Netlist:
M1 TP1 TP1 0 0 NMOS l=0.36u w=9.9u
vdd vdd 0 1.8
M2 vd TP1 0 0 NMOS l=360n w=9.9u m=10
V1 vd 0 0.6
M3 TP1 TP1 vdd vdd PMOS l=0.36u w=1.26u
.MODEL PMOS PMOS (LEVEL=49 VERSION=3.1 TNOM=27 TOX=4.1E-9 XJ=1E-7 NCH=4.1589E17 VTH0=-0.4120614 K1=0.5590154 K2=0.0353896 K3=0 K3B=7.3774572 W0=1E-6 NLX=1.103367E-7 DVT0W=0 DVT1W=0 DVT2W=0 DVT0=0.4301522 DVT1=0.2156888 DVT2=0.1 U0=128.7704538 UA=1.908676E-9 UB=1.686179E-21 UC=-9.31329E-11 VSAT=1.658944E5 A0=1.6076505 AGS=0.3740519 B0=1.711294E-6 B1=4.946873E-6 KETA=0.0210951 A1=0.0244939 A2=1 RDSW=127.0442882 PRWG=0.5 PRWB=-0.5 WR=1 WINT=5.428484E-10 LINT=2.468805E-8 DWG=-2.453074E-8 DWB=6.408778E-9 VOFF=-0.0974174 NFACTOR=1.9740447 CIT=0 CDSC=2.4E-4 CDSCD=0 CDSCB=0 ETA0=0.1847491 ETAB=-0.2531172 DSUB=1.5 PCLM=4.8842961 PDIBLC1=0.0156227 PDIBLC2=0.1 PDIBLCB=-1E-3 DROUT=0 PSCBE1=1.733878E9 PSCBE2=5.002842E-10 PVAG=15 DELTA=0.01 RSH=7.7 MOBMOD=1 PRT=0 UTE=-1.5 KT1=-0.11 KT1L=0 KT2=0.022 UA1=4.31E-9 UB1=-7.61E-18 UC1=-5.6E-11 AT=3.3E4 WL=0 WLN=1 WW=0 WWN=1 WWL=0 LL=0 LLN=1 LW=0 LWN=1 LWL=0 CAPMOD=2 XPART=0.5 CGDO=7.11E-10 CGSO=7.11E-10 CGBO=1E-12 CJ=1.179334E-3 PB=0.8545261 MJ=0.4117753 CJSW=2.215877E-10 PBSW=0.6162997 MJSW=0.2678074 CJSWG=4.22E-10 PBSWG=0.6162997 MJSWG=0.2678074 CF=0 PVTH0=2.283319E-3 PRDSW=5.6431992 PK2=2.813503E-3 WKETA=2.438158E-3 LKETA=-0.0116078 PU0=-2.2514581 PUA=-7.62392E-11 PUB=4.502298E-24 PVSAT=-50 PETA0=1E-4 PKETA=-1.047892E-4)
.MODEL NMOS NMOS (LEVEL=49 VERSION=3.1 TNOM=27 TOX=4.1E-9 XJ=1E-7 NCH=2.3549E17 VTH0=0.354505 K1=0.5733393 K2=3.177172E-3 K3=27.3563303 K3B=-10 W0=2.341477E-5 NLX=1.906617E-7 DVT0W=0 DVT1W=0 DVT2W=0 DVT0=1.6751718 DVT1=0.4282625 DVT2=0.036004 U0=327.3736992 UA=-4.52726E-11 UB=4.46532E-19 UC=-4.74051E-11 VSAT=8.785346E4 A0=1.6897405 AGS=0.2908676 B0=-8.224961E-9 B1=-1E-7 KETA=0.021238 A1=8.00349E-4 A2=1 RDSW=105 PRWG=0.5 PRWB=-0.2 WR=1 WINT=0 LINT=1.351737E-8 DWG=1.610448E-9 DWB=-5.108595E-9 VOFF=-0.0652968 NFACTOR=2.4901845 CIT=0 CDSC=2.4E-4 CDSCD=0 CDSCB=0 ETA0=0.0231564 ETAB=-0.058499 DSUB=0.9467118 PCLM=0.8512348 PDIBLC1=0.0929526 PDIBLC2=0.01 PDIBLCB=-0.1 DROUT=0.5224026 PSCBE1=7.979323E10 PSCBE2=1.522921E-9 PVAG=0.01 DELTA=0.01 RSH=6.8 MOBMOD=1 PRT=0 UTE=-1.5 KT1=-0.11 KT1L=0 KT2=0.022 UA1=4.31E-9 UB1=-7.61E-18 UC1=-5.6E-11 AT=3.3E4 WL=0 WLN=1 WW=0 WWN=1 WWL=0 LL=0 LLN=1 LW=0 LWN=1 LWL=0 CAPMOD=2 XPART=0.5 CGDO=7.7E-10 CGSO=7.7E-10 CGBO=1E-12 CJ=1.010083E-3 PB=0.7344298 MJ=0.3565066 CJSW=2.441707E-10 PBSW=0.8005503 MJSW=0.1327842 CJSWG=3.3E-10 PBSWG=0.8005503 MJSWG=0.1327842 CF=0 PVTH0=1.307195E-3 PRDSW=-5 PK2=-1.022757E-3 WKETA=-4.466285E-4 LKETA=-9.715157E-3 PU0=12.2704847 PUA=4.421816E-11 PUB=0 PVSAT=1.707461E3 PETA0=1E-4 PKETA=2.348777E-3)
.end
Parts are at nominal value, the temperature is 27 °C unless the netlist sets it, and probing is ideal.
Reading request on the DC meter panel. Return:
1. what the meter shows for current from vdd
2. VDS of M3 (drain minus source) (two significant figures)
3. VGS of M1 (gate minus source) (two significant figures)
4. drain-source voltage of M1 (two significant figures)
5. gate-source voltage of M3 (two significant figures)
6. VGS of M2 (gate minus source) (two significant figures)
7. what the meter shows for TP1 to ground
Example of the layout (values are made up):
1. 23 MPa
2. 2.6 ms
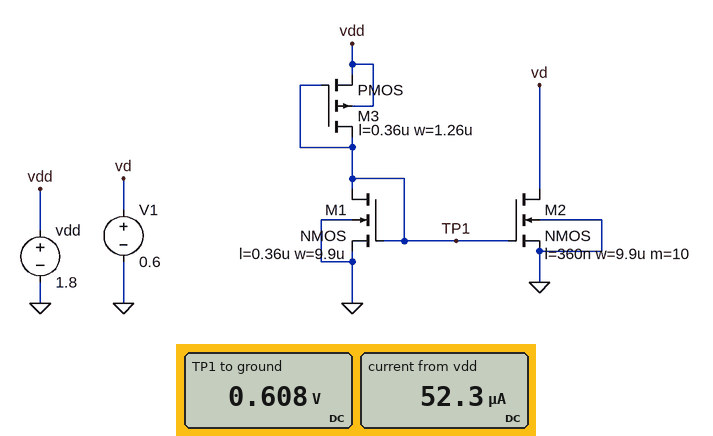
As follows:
1. 52.3 µA
2. -1.2 V
3. 610 mV
4. 610 mV
5. -1.2 V
6. 610 mV
7. 0.608 V
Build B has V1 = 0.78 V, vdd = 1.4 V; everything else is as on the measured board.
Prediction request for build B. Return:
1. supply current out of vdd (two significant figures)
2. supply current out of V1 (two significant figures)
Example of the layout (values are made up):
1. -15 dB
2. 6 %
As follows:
1. 17 µA
2. 180 µA
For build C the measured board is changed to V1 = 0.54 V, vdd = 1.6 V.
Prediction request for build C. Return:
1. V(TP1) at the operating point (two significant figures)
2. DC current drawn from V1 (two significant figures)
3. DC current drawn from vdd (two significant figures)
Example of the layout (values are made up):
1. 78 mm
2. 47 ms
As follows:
1. 580 mV
2. 320 µA
3. 32 µA
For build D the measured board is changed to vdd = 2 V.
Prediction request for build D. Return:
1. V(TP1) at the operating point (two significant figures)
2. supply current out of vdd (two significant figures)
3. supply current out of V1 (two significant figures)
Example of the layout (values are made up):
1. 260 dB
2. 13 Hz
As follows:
1. 630 mV
2. 76 µA
3. 760 µA
